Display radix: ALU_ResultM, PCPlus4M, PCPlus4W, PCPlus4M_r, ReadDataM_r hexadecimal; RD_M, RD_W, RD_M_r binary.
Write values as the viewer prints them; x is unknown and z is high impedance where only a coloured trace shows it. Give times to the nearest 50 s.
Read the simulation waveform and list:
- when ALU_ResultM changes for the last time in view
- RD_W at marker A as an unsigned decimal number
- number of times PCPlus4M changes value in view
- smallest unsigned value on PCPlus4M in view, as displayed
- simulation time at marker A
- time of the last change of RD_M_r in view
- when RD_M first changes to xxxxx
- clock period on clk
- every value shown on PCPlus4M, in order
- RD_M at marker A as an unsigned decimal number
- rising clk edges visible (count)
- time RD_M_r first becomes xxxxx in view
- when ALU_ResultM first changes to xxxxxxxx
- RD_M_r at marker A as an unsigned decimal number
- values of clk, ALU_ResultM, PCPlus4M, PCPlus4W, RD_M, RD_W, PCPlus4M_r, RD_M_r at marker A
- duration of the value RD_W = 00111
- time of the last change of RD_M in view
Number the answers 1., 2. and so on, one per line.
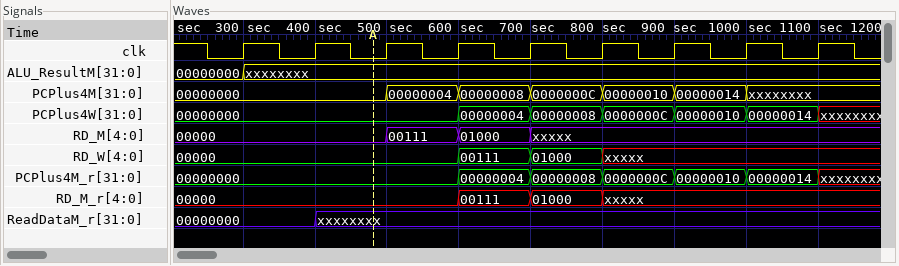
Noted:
1. 300 s
2. 0
3. 6
4. 00000000
5. 500 s
6. 800 s
7. 700 s
8. 100 s
9. 00000000, 00000004, 00000008, 0000000C, 00000010, 00000014, xxxxxxxx
10. 0
11. 9
12. 800 s
13. 300 s
14. 0
15. clk=0, ALU_ResultM=xxxxxxxx, PCPlus4M=00000000, PCPlus4W=00000000, RD_M=00000, RD_W=00000, PCPlus4M_r=00000000, RD_M_r=00000
16. 100 s
17. 700 s
